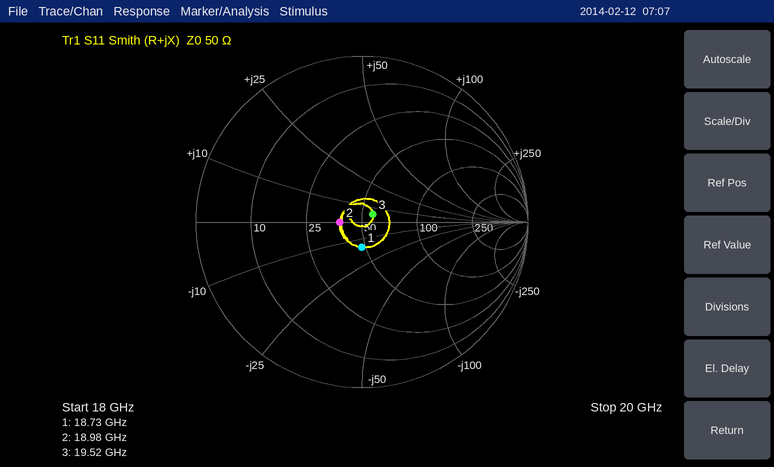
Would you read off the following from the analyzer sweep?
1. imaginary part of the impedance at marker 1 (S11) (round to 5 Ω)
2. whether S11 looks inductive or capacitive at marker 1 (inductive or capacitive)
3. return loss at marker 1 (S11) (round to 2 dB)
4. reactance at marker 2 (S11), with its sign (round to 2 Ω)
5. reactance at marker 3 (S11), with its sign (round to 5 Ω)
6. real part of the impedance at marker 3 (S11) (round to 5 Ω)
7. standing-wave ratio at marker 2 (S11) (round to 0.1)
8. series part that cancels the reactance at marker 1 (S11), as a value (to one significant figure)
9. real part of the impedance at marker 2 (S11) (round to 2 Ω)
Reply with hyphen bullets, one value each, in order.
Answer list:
- -15 Ω
- capacitive
- 16 dB
- 0 Ω
- +5 Ω
- 55 Ω
- 1.3
- 100 pH
- 38 Ω
